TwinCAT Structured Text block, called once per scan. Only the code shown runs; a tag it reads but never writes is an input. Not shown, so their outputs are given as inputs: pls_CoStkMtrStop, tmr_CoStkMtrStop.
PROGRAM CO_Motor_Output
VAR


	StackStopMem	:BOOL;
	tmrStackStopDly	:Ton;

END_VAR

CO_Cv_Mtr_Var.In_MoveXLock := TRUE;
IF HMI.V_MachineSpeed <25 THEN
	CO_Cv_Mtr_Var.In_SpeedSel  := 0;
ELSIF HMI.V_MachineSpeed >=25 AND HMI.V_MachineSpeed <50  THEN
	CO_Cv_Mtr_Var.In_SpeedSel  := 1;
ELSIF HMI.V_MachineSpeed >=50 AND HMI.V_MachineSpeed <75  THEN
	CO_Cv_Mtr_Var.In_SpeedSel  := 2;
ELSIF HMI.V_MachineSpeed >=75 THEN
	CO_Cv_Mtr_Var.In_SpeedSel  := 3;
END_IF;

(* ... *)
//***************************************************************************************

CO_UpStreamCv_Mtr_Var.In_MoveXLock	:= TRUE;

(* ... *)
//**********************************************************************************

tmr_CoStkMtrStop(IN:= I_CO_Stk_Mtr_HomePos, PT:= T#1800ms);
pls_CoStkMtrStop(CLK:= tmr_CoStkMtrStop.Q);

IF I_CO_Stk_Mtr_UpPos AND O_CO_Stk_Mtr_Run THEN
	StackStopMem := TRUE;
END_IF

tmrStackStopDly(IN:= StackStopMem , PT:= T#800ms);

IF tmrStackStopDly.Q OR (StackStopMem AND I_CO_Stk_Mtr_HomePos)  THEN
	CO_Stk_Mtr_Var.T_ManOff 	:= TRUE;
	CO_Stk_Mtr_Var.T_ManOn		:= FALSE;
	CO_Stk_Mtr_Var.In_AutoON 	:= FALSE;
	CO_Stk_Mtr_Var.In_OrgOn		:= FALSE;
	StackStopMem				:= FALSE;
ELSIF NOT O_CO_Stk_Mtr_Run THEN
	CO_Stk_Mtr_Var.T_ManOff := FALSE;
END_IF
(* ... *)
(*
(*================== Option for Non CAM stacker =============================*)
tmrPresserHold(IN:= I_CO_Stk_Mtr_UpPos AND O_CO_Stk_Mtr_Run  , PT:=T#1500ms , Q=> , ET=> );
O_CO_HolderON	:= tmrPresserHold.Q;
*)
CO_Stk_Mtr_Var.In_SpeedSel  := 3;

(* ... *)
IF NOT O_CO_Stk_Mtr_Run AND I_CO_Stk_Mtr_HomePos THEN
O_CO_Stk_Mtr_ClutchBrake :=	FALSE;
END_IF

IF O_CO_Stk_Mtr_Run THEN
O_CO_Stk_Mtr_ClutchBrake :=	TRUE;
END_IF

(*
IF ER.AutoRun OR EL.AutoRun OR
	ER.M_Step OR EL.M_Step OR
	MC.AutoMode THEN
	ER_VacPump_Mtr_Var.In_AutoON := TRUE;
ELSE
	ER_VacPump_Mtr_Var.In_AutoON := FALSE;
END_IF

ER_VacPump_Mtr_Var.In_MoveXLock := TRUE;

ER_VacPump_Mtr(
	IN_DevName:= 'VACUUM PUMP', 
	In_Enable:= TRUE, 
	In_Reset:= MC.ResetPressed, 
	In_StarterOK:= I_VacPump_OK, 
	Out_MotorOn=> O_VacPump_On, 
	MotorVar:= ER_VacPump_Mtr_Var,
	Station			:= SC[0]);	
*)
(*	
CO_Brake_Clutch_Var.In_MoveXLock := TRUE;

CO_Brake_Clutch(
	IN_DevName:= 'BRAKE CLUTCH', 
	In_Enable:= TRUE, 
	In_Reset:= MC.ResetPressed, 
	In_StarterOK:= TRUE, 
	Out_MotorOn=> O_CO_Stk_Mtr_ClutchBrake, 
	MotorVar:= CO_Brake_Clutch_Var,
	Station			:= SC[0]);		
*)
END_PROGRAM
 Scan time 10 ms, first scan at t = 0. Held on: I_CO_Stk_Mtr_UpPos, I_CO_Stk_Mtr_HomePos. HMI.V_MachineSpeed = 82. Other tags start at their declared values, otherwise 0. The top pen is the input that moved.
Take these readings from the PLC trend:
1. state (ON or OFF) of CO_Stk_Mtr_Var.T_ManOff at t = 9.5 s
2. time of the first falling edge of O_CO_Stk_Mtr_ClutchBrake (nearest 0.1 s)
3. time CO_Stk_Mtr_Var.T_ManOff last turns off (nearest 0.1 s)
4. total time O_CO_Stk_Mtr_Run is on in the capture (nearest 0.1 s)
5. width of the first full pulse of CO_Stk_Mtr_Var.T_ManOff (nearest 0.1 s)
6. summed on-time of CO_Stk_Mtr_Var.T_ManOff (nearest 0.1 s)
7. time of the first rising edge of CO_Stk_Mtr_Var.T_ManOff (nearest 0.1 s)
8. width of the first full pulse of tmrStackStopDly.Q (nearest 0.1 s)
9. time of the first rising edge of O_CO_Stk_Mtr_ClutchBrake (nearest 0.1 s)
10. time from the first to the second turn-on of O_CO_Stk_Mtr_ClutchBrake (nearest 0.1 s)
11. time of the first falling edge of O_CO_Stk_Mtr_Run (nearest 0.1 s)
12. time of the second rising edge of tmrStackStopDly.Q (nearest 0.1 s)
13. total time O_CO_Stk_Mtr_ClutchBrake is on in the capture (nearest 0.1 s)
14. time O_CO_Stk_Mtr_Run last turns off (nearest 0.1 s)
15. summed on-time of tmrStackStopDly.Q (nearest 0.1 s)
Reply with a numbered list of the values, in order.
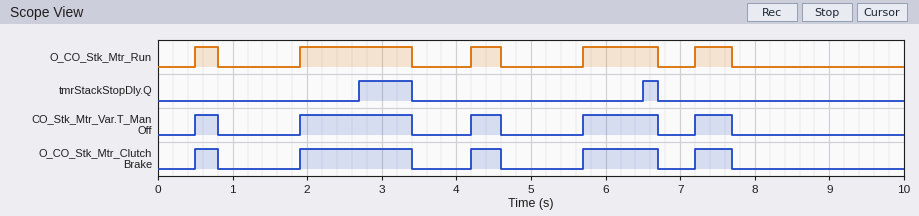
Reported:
1. OFF
2. 0.8 s
3. 7.7 s
4. 3.7 s
5. 0.3 s
6. 3.7 s
7. 0.5 s
8. 0.7 s
9. 0.5 s
10. 1.4 s
11. 0.8 s
12. 6.5 s
13. 3.7 s
14. 7.7 s
15. 0.9 s
